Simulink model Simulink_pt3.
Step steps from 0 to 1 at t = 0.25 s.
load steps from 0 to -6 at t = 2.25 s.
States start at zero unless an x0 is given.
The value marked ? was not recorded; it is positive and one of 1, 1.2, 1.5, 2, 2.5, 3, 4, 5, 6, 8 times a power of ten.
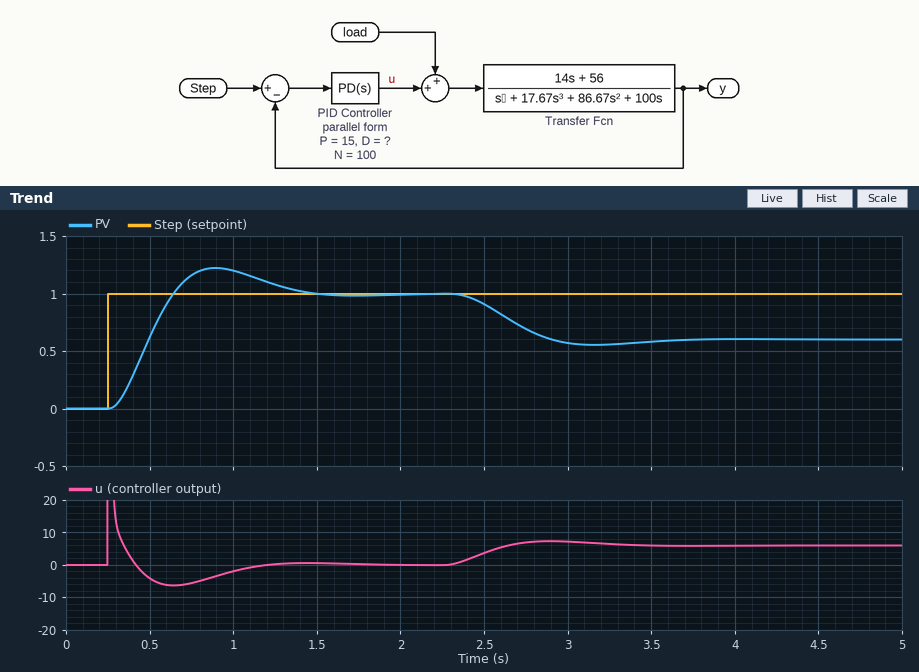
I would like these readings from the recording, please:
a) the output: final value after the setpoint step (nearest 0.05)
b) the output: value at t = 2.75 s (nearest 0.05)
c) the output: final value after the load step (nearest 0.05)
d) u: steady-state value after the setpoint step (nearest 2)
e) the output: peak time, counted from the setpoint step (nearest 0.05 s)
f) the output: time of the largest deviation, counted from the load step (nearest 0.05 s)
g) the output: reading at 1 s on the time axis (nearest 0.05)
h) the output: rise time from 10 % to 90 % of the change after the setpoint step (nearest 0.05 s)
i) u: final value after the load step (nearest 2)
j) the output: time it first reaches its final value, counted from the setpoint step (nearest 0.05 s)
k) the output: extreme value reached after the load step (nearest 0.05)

1.00
0.70
0.60
0
0.65 s
0.90 s
1.20
0.25 s
6
0.40 s
0.55
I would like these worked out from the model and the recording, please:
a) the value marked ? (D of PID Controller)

3
